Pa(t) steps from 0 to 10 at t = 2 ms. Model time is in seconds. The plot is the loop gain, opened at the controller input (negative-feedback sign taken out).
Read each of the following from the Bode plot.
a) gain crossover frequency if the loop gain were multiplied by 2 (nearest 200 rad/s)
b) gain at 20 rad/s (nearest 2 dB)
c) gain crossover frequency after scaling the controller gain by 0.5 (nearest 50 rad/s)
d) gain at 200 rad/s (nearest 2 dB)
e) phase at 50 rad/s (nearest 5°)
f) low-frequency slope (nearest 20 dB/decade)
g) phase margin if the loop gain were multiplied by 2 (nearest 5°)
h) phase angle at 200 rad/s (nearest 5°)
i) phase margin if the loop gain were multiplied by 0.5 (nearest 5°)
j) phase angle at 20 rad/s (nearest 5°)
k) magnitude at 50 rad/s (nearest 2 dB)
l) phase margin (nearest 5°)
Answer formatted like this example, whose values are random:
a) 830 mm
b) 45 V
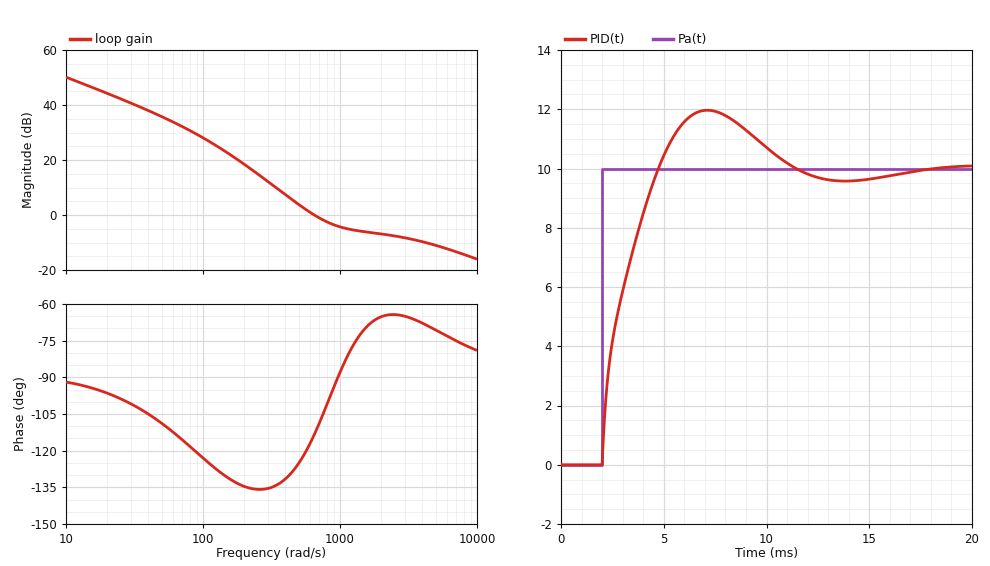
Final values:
a) 1400 rad/s
b) 44 dB
c) 450 rad/s
d) 18 dB
e) -110°
f) -20 dB/decade
g) 110°
h) -135°
i) 50°
j) -95°
k) 36 dB
l) 65°
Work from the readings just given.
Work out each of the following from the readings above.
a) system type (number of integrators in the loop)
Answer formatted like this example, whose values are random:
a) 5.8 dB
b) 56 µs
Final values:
a) 1
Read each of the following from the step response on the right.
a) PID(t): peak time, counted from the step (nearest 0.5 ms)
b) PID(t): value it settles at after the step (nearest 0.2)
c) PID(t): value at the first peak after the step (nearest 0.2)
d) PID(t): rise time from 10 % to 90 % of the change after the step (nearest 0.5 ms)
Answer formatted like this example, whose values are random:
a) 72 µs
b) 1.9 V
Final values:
a) 5.0 ms
b) 10.0
c) 12.0
d) 2.0 ms
